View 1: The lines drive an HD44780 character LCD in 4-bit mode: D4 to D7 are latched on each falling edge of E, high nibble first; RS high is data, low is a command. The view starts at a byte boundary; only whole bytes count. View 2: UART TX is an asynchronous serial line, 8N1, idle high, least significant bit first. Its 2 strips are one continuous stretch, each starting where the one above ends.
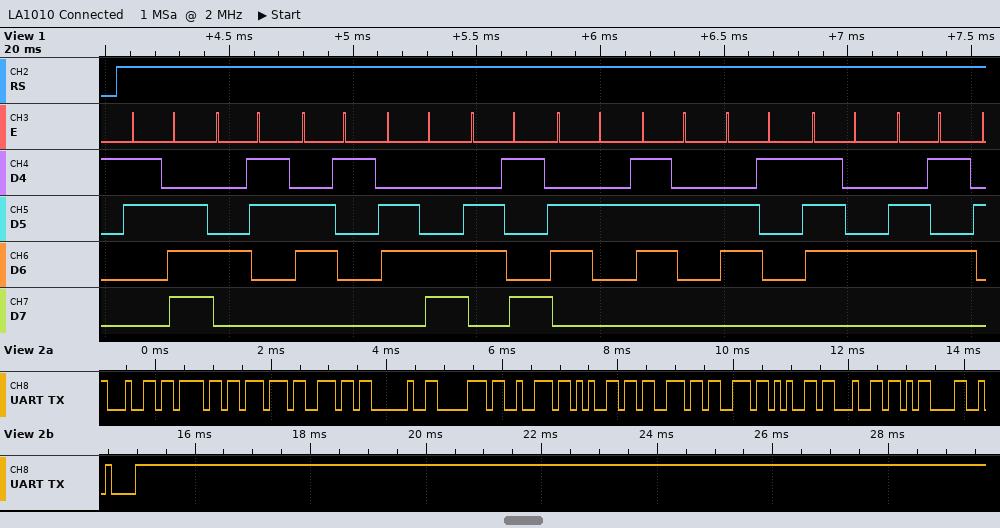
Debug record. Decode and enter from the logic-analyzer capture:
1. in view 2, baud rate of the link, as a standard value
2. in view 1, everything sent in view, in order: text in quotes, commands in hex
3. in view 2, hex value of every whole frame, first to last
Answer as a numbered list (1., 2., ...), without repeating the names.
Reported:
1. 9600 baud
2. ">Calibrate"
3. 0x64 0x6F 0x77 0x6E 0x20 0x70 0x72 0x65 0x73 0x73 0x65 0x64 0x0D 0x0A
